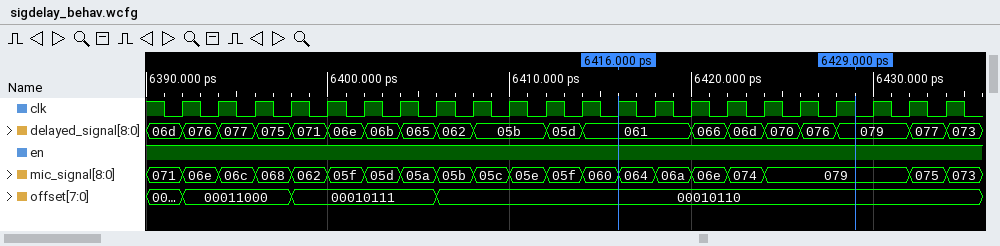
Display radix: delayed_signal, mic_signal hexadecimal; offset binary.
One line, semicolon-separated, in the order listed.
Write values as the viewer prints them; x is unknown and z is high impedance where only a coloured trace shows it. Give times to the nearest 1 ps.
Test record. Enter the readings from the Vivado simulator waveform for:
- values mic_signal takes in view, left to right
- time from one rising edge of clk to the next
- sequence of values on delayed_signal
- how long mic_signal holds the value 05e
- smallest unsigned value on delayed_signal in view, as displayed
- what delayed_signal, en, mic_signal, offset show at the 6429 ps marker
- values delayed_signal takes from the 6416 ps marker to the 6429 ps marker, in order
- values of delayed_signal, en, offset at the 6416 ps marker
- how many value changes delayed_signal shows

071, 06e, 06c, 068, 062, 05f, 05d, 05a, 05b, 05c, 05e, 05f, 060, 064, 06a, 06e, 074, 079, 075, 073; 2 ps; 06d, 076, 077, 075, 071, 06e, 06b, 065, 062, 05b, 05d, 061, 066, 06d, 070, 076, 079, 077, 073; 2 ps; 05b; delayed_signal=079, en=1, mic_signal=079, offset=00010110; 061, 066, 06d, 070, 076, 079; delayed_signal=061, en=1, offset=00010110; 18
